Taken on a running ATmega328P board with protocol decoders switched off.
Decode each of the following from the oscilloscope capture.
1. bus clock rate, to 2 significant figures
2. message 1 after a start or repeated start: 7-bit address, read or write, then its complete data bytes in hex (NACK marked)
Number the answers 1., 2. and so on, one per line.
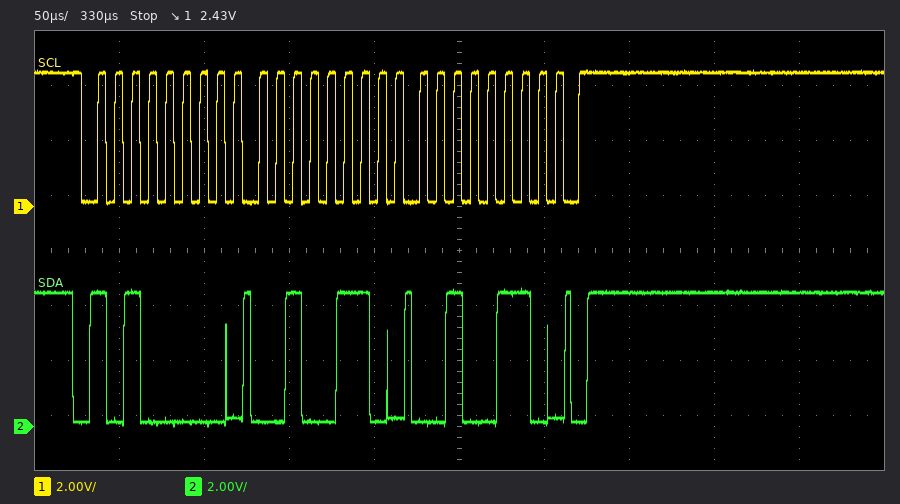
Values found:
1. 100 kHz
2. 0x50 write: 26 26
